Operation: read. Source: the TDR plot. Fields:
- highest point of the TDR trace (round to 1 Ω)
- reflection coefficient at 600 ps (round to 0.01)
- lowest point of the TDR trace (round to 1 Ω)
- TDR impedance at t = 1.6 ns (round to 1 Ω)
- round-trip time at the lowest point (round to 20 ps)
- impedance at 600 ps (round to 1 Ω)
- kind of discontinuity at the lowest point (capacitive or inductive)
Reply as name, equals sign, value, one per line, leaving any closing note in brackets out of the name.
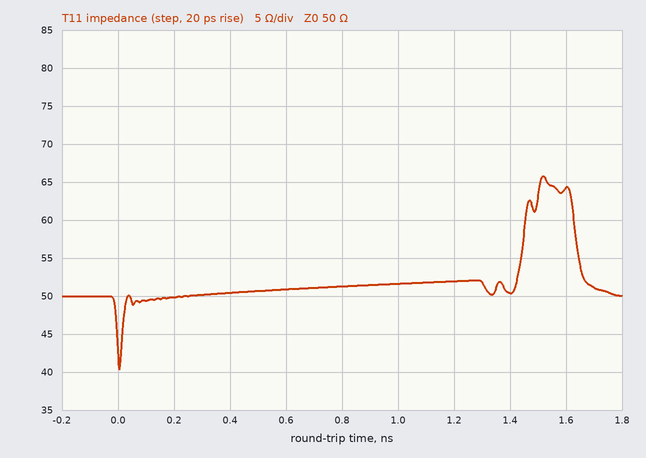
highest point of the TDR trace = 66 Ω
reflection coefficient at 600 ps = +0.01
lowest point of the TDR trace = 40 Ω
TDR impedance at t = 1.6 ns = 64 Ω
round-trip time at the lowest point = 0 ps
impedance at 600 ps = 51 Ω
kind of discontinuity at the lowest point = capacitive
